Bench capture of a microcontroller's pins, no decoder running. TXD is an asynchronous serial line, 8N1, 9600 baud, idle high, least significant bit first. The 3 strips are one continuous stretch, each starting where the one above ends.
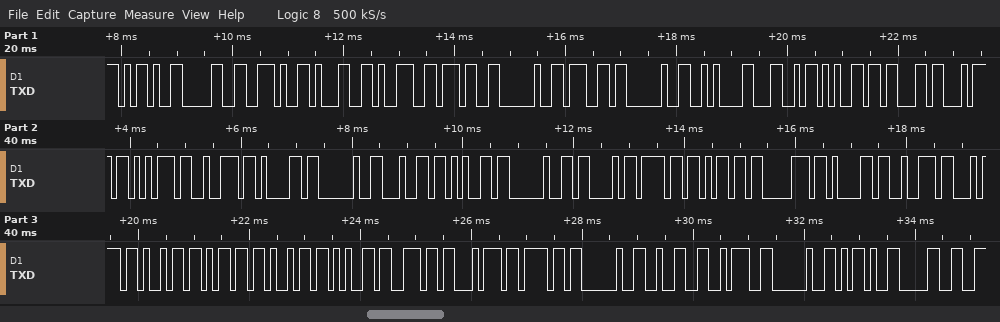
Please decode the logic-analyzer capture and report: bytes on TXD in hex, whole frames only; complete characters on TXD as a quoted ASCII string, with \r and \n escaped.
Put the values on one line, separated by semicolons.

2D 30 2E 31 39 37 20 67 20 0A 4C 65 63 74 75 72 61 20 64 65 20 43 6F 6D 70 61 72 74 69 6D 69 65 6E 74 6F 20 32 3A 20 2D 30; "-0.197 g \nLectura de Compartimiento 2: -0"
